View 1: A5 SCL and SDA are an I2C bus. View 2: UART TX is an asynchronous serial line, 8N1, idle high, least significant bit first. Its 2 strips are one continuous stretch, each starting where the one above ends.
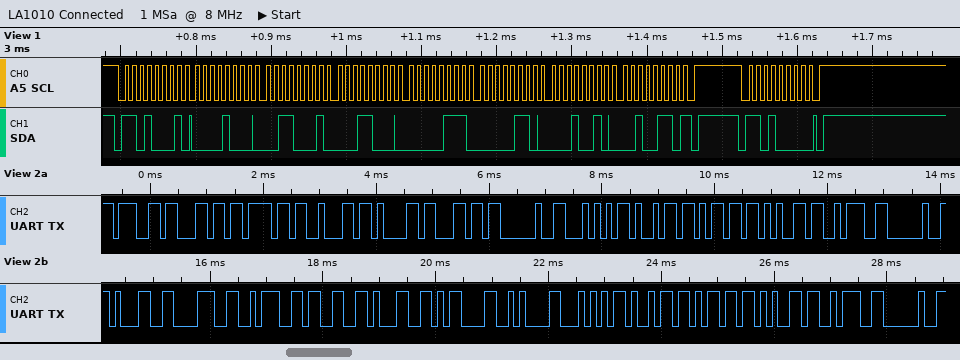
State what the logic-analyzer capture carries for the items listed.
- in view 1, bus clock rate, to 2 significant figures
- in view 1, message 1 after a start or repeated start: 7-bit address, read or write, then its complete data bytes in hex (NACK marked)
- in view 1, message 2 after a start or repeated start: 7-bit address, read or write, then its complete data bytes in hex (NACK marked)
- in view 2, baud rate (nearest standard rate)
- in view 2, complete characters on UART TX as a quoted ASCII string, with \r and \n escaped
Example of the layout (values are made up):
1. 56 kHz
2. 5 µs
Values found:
1. 100 kHz
2. 0x68 read: 08 31 18 07 06 12 26 NACK
3. 0x68 write
4. 9600 baud
5. "global Time: 18:31\r\nTime: "
